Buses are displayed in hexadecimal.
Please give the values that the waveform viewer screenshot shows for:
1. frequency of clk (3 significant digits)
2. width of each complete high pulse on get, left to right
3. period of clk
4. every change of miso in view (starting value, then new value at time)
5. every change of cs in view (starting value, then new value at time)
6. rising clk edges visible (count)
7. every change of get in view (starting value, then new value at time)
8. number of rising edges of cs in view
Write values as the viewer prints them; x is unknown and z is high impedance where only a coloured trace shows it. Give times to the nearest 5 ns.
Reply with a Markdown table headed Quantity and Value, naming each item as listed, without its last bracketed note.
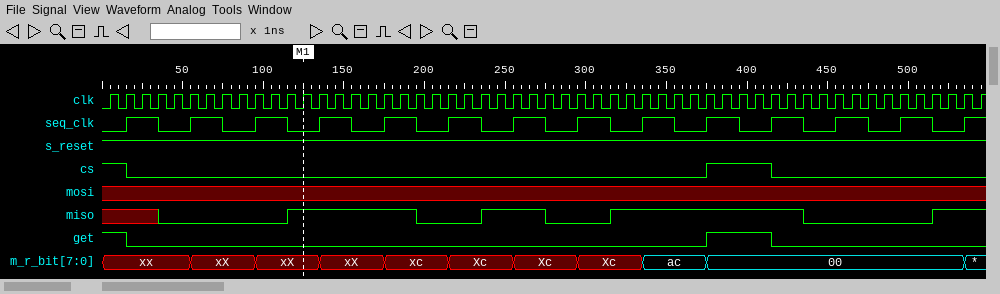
| Quantity | Value |
|---|---|
| frequency of clk | 100 MHz |
| width of each complete high pulse on get, left to right | 40 ns |
| period of clk | 10 ns |
| every change of miso in view | x, 0 at 35 ns, 1 at 115 ns, 0 at 195 ns, 1 at 235 ns, 0 at 275 ns, 1 at 315 ns, 0 at 435 ns, 1 at 515 ns |
| every change of cs in view | 1, 0 at 15 ns, 1 at 375 ns, 0 at 415 ns |
| rising clk edges visible | 55 |
| every change of get in view | 1, 0 at 15 ns, 1 at 375 ns, 0 at 415 ns |
| number of rising edges of cs in view | 1 |
